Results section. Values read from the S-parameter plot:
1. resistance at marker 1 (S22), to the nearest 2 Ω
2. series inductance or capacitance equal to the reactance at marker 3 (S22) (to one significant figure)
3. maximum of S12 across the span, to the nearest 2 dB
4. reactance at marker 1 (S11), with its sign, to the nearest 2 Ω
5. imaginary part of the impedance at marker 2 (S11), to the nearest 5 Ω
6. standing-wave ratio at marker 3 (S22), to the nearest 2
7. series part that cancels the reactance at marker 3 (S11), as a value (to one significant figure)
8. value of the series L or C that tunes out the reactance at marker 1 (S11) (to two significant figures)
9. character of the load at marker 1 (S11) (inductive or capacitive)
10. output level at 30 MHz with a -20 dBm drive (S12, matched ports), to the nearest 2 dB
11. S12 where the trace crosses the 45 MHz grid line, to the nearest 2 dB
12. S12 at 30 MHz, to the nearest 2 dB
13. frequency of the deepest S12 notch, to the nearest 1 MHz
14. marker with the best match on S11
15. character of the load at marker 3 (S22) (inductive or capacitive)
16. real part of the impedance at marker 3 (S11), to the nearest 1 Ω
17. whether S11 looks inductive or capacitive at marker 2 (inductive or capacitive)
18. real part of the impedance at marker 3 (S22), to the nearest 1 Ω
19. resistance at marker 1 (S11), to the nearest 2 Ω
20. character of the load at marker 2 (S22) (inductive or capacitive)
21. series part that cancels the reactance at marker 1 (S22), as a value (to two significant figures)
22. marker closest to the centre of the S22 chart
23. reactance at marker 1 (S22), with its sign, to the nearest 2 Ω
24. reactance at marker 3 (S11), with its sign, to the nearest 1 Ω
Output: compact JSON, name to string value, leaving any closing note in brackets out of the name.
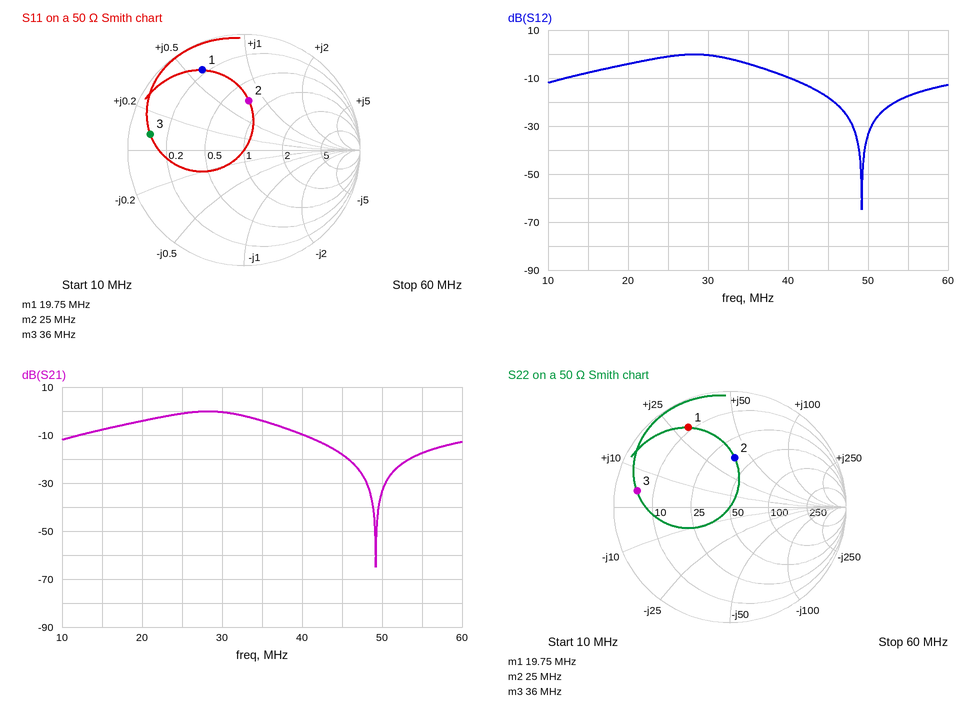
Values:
{"resistance at marker 1 (S22), to the nearest 2 Ω": "8 Ω", "series inductance or capacitance equal to the reactance at marker 3 (S22)": "20 nH", "maximum of S12 across the span, to the nearest 2 dB": "0 dB", "reactance at marker 1 (S11), with its sign, to the nearest 2 Ω": "+30 Ω", "imaginary part of the impedance at marker 2 (S11), to the nearest 5 Ω": "+40 Ω", "standing-wave ratio at marker 3 (S22), to the nearest 2": "10", "series part that cancels the reactance at marker 3 (S11), as a value": "1 nF", "value of the series L or C that tunes out the reactance at marker 1 (S11)": "270 pF", "character of the load at marker 1 (S11)": "inductive", "output level at 30 MHz with a -20 dBm drive (S12, matched ports), to the nearest 2 dB": "-20 dBm", "S12 where the trace crosses the 45 MHz grid line, to the nearest 2 dB": "-18 dB", "S12 at 30 MHz, to the nearest 2 dB": "0 dB", "frequency of the deepest S12 notch, to the nearest 1 MHz": "49 MHz", "marker with the best match on S11": "marker 2", "character of the load at marker 3 (S22)": "inductive", "real part of the impedance at marker 3 (S11), to the nearest 1 Ω": "5 Ω", "whether S11 looks inductive or capacitive at marker 2": "inductive", "real part of the impedance at marker 3 (S22), to the nearest 1 Ω": "5 Ω", "resistance at marker 1 (S11), to the nearest 2 Ω": "8 Ω", "character of the load at marker 2 (S22)": "inductive", "series part that cancels the reactance at marker 1 (S22), as a value": "270 pF", "marker closest to the centre of the S22 chart": "marker 2", "reactance at marker 1 (S22), with its sign, to the nearest 2 Ω": "+30 Ω", "reactance at marker 3 (S11), with its sign, to the nearest 1 Ω": "+4 Ω"}
